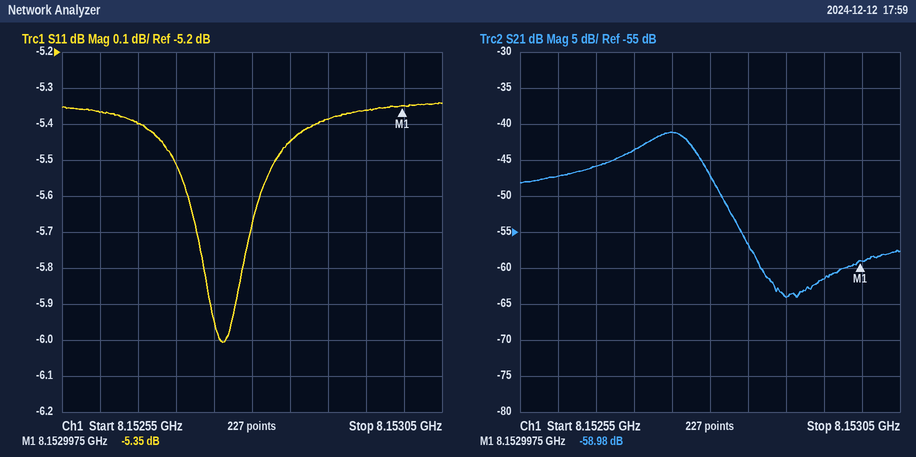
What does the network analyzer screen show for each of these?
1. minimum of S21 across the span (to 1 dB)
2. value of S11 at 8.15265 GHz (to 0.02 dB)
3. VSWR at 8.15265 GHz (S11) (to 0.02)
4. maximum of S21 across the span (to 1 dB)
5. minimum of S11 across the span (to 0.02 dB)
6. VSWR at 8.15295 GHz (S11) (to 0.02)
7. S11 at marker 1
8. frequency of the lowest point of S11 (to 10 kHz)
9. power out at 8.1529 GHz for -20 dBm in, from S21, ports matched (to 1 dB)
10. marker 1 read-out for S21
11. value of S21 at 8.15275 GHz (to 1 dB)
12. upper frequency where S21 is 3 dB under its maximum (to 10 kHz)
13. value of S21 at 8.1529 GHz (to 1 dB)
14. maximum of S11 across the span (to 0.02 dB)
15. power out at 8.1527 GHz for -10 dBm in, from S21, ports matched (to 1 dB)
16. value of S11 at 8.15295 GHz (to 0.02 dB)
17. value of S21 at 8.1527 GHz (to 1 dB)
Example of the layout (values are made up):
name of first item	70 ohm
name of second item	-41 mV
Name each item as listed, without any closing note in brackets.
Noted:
minimum of S21 across the span	-64 dB
value of S11 at 8.15265 GHz	-5.40 dB
VSWR at 8.15265 GHz (S11)	3.32
maximum of S21 across the span	-41 dB
minimum of S11 across the span	-6.00 dB
VSWR at 8.15295 GHz (S11)	3.34
S11 at marker 1	-5.35 dB
frequency of the lowest point of S11	8.15276 GHz
power out at 8.1529 GHz for -20 dBm in, from S21, ports matched	-84 dBm
marker 1 read-out for S21	-58.98 dB
value of S21 at 8.15275 GHz	-41 dB
upper frequency where S21 is 3 dB under its maximum	8.15278 GHz
value of S21 at 8.1529 GHz	-64 dB
maximum of S11 across the span	-5.34 dB
power out at 8.1527 GHz for -10 dBm in, from S21, ports matched	-54 dBm
value of S11 at 8.15295 GHz	-5.36 dB
value of S21 at 8.1527 GHz	-44 dB
